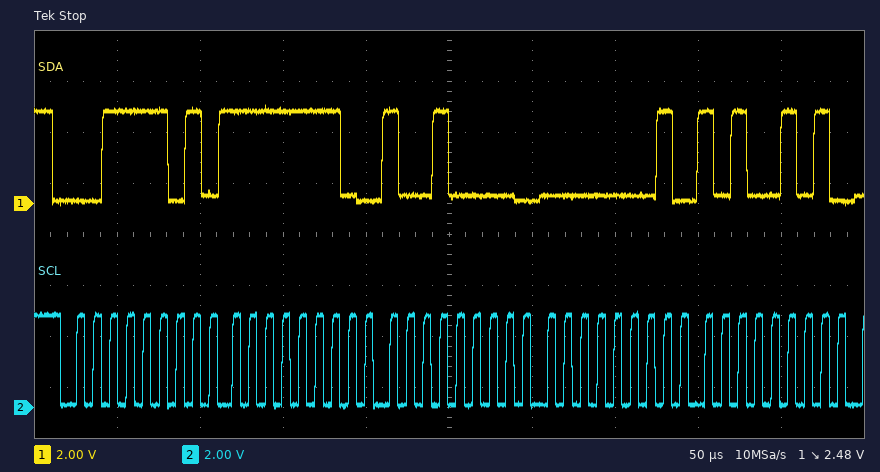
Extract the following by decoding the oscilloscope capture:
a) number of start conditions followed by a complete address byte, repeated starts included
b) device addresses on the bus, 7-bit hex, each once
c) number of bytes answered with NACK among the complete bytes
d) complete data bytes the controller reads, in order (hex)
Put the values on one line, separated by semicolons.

1; 0x1E; 0; FE 90 01 A5
